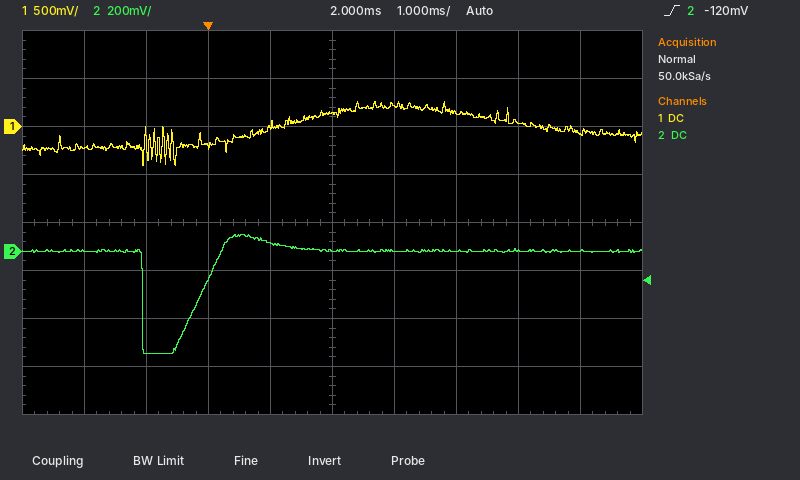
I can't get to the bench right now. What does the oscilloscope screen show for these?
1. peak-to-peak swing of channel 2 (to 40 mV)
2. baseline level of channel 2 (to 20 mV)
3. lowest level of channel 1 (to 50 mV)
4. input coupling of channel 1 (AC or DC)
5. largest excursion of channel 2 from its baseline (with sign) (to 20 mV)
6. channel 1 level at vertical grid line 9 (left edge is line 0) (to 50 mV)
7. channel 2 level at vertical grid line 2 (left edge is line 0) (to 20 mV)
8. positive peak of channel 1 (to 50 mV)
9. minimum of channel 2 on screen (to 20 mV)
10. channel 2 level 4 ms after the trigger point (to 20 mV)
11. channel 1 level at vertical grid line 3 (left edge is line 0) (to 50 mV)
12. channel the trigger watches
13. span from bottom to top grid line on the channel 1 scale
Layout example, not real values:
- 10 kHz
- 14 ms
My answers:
- 480 mV
- 0 mV
- -400 mV
- DC
- -420 mV
- -50 mV
- -420 mV
- 250 mV
- -420 mV
- 0 mV
- -200 mV
- channel 2
- 4 V
